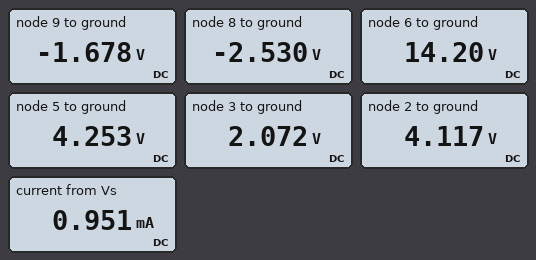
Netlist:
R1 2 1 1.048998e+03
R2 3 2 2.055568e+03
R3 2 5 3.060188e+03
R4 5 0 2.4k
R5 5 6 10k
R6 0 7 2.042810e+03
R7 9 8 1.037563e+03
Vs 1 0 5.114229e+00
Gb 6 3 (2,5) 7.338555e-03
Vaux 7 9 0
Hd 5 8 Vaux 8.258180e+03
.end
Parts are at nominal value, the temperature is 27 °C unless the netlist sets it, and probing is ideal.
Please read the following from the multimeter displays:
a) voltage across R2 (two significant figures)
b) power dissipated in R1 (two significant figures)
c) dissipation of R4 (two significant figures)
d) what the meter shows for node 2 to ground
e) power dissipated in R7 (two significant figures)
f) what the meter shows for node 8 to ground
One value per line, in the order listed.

2.0 V
950 µW
7.5 mW
4.117 V
700 µW
-2.530 V
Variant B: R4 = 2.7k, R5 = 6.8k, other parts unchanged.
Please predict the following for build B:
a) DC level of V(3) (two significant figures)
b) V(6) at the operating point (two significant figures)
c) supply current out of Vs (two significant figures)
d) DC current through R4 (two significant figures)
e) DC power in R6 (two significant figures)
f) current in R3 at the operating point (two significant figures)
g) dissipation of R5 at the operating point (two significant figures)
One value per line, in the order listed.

2.6 V
10 V
780 µA
1.6 mA
1.5 mW
36 µA
4.5 mW
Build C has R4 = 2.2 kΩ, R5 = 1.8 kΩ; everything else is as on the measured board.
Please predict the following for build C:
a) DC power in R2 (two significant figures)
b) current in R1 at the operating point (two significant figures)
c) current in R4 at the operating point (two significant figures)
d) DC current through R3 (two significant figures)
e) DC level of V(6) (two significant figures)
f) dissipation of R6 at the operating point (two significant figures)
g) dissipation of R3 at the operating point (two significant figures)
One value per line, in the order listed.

2.6 mW
1.1 mA
1.9 mA
50 µA
6.2 V
1.3 mW
7.8 µW
